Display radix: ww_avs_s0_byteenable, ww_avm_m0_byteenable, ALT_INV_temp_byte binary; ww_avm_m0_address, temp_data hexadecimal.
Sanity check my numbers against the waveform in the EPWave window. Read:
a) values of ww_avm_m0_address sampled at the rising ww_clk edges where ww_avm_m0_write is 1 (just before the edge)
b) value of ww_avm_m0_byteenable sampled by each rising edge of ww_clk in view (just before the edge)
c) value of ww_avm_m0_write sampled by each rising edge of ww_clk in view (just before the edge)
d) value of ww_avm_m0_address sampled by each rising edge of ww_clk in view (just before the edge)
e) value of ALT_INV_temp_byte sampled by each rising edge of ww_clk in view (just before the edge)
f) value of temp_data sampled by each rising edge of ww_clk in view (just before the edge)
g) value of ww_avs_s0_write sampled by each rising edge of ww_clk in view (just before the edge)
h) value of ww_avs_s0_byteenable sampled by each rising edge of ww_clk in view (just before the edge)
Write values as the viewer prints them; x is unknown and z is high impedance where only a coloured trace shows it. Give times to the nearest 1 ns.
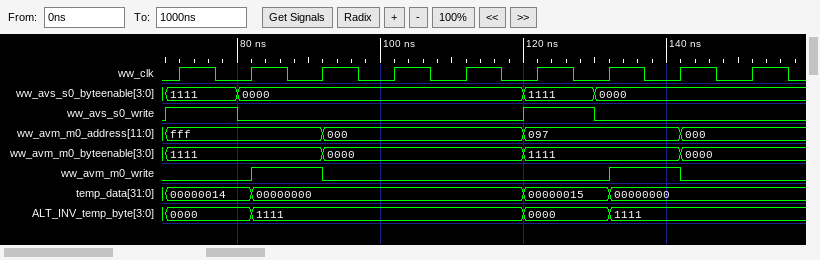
fff, 097
1111, 1111, 1111, 0000, 0000, 1111, 1111, 1111, 0000
0 0 1 0 0 0 0 1 0
fff, fff, fff, 000, 000, 097, 097, 097, 000
0000, 0000, 1111, 1111, 1111, 0000, 0000, 1111, 1111
00000014, 00000014, 00000000, 00000000, 00000000, 00000015, 00000015, 00000000, 00000000
1 0 0 0 0 1 0 0 0
1111, 0000, 0000, 0000, 0000, 1111, 0000, 0000, 0000
